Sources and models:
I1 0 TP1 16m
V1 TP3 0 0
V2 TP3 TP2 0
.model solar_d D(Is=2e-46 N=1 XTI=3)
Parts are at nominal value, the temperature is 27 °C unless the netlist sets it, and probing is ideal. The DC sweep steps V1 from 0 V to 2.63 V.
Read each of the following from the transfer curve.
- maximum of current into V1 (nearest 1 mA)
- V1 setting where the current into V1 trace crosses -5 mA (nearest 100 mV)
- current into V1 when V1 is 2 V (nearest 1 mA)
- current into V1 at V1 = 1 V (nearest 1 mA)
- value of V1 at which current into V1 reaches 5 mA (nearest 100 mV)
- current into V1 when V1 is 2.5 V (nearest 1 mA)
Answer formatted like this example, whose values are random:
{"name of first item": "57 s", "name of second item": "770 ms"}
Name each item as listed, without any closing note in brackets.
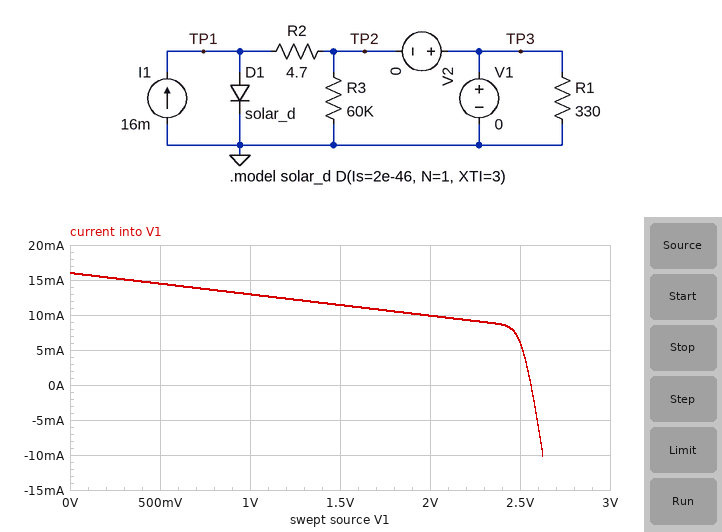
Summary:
{"maximum of current into V1": "16 mA", "V1 setting where the current into V1 trace crosses -5 mA": "2.6 V", "current into V1 when V1 is 2 V": "10 mA", "current into V1 at V1 = 1 V": "13 mA", "value of V1 at which current into V1 reaches 5 mA": "2.5 V", "current into V1 when V1 is 2.5 V": "6 mA"}
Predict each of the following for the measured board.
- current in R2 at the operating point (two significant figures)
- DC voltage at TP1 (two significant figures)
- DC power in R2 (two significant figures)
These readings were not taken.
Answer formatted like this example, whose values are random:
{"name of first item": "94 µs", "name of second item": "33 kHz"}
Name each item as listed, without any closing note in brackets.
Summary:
{"current in R2 at the operating point": "16 mA", "DC voltage at TP1": "75 mV", "DC power in R2": "1.2 mW"}
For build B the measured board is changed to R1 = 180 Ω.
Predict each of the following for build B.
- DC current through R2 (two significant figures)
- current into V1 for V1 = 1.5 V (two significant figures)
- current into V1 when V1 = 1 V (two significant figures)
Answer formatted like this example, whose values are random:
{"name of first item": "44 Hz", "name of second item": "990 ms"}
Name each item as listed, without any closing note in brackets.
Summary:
{"DC current through R2": "16 mA", "current into V1 for V1 = 1.5 V": "7.6 mA", "current into V1 when V1 = 1 V": "10 mA"}
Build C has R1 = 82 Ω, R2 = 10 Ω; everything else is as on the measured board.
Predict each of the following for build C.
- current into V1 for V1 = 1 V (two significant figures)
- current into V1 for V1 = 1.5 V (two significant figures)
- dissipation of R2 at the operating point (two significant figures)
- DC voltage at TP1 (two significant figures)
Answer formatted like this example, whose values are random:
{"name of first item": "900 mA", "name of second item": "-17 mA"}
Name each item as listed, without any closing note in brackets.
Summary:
{"current into V1 for V1 = 1 V": "3.8 mA", "current into V1 for V1 = 1.5 V": "-2.3 mA", "dissipation of R2 at the operating point": "2.6 mW", "DC voltage at TP1": "160 mV"}
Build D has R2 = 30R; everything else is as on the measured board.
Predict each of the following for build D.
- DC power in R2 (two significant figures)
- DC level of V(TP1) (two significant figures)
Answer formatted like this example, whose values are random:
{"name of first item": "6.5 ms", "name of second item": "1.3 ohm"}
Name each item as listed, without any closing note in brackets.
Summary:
{"DC power in R2": "7.7 mW", "DC level of V(TP1)": "480 mV"}
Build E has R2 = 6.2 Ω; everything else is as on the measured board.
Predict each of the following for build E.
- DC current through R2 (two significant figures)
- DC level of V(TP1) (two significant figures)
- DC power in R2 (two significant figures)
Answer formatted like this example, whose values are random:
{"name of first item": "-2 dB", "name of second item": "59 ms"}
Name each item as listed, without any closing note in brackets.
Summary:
{"DC current through R2": "16 mA", "DC level of V(TP1)": "99 mV", "DC power in R2": "1.6 mW"}
